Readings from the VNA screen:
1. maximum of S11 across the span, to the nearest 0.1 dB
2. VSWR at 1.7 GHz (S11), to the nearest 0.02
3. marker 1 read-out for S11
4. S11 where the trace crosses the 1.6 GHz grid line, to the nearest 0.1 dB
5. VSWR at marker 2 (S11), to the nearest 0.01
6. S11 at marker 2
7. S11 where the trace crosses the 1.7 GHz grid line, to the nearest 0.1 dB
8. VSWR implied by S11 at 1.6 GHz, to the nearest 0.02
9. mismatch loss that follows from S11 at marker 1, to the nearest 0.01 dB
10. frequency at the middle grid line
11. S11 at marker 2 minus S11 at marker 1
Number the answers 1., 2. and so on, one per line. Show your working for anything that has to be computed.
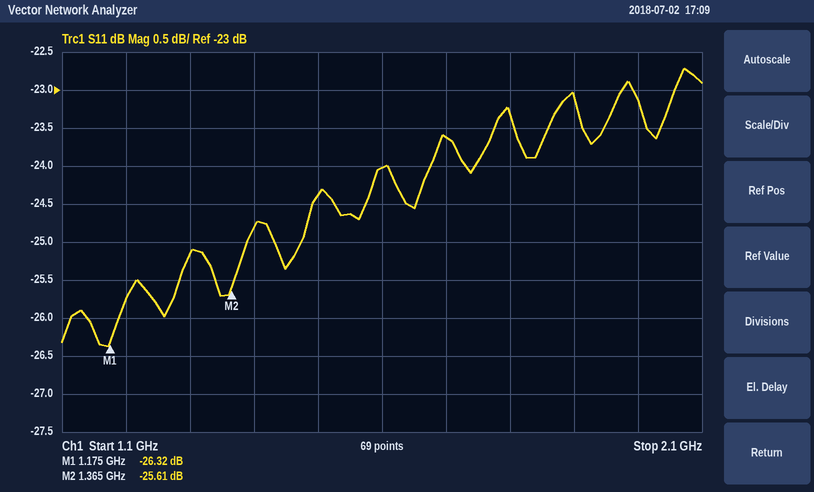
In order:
1. -22.7 dB
2. |Γ| = 10^(-23.6/20) = 0.0661; VSWR = (1 + 0.0661)/(1 − 0.0661) ≈ 1.14
3. -26.32 dB
4. -24.0 dB
5. (1 + 0.0524)/(1 − 0.0524) ≈ 1.11
6. -25.61 dB
7. -23.6 dB
8. |Γ| = 10^(-24/20) = 0.0631; VSWR = (1 + 0.0631)/(1 − 0.0631) ≈ 1.13, so 1.14 to the nearest 0.02
9. −10 log10(1 − 10^(-26.32/10)) ≈ 0.01 dB
10. 1.6 GHz
11. -25.61 − (-26.32) = 0.71 dB
